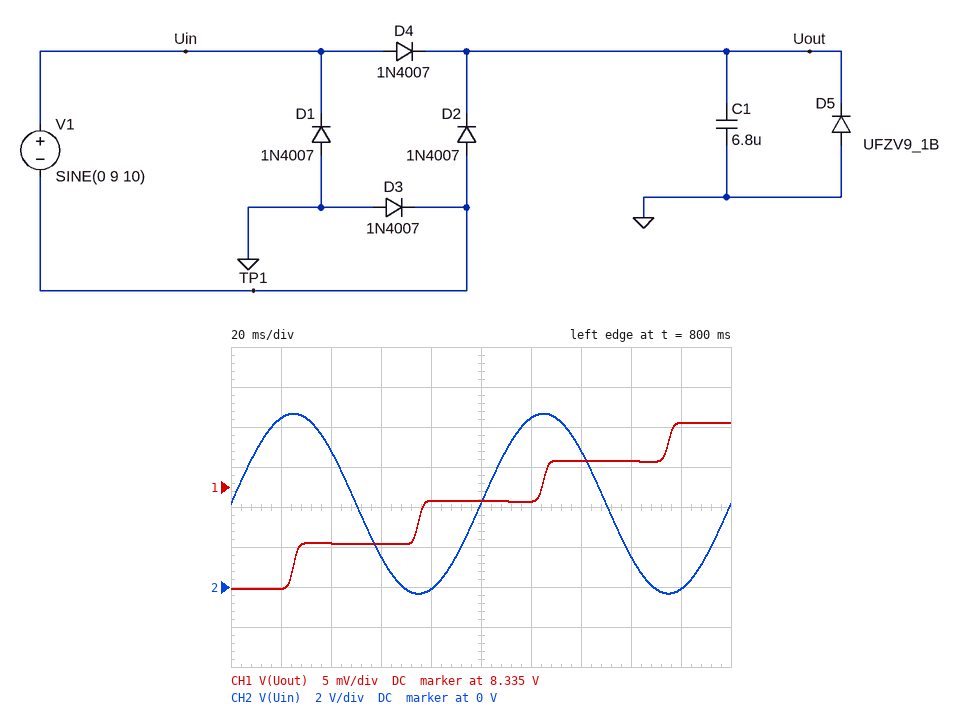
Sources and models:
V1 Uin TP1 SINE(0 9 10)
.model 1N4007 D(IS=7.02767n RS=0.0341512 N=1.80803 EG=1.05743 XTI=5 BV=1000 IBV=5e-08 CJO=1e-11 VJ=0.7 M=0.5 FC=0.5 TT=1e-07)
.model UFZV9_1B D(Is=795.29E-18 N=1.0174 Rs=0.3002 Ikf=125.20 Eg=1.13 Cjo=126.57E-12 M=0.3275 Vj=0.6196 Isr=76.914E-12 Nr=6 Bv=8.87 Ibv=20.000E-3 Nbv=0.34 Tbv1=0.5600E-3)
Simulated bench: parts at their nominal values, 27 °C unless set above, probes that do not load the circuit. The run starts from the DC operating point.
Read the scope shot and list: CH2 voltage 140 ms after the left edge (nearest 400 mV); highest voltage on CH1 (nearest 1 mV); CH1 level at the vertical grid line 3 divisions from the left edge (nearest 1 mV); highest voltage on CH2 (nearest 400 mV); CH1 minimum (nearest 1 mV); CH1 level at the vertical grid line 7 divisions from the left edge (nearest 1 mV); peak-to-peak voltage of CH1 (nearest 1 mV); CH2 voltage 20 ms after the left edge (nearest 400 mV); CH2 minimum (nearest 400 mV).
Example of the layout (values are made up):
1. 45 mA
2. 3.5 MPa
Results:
1. 6.8 V
2. 8.343 V
3. 8.328 V
4. 8.8 V
5. 8.322 V
6. 8.338 V
7. 21 mV
8. 8.4 V
9. -400 mV
